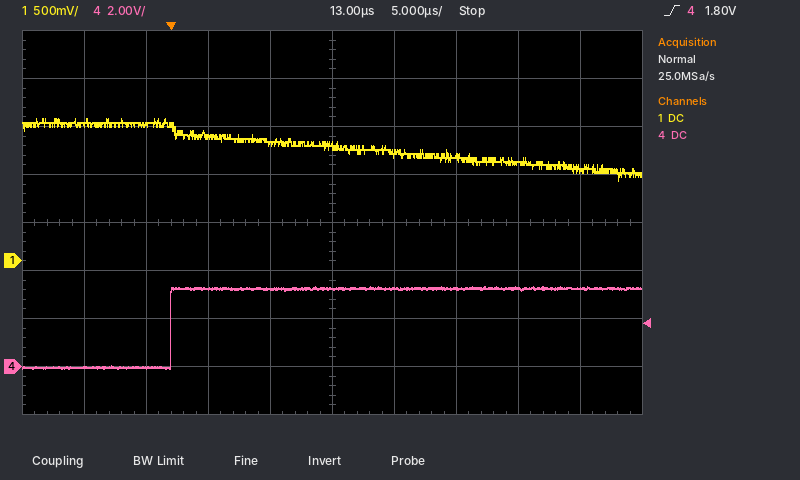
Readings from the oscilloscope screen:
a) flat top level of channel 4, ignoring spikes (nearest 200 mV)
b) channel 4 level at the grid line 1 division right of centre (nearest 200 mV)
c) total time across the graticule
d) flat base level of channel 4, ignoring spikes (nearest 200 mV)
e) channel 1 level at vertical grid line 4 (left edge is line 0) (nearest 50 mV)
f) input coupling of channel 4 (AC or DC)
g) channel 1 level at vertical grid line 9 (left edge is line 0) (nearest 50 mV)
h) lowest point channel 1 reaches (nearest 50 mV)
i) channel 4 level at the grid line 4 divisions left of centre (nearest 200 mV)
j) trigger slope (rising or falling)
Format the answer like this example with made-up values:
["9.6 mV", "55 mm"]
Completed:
["3.2 V", "3.2 V", "50 µs", "0.0 V", "1.20 V", "DC", "950 mV", "850 mV", "0.0 V", "rising"]
